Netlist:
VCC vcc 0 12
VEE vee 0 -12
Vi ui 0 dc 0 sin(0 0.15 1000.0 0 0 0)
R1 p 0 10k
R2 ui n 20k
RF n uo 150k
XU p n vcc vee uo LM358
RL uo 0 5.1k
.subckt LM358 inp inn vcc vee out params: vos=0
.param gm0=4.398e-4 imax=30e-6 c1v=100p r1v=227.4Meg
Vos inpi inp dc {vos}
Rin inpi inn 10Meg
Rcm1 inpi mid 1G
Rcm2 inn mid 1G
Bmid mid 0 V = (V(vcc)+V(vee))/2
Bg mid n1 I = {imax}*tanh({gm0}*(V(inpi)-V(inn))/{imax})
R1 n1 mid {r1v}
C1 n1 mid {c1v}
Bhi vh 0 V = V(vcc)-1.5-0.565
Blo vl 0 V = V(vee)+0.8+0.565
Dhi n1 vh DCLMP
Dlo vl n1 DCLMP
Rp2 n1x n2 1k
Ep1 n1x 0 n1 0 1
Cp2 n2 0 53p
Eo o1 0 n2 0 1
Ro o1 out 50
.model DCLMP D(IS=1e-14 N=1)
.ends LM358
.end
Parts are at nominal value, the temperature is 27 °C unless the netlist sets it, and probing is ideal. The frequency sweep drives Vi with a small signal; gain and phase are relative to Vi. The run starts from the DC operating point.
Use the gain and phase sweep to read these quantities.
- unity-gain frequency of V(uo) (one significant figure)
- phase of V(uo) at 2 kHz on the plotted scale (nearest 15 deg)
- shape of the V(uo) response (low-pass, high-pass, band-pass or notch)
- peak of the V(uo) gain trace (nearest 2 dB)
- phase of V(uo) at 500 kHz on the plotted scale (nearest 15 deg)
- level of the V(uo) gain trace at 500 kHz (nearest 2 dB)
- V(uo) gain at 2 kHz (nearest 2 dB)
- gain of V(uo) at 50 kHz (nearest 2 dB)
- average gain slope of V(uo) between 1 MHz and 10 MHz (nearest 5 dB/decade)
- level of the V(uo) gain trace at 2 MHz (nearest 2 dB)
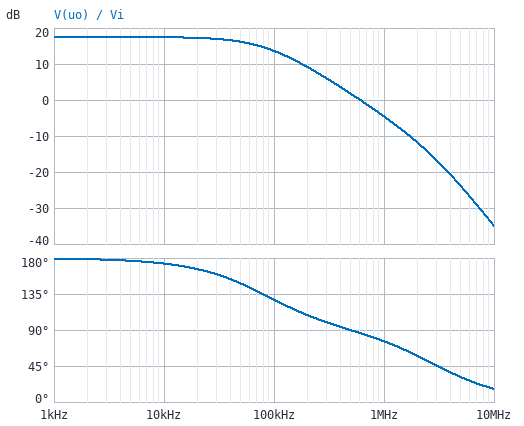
600 kHz
180 deg
low-pass
18 dB
90 deg
2 dB
18 dB
16 dB
-30 dB/decade
-12 dB
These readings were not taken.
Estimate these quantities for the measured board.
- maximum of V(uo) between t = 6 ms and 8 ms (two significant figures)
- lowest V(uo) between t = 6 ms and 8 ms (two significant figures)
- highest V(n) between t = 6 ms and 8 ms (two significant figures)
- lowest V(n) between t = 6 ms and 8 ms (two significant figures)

1.1 V
-1.1 V
1.6 mV
-1.6 mV
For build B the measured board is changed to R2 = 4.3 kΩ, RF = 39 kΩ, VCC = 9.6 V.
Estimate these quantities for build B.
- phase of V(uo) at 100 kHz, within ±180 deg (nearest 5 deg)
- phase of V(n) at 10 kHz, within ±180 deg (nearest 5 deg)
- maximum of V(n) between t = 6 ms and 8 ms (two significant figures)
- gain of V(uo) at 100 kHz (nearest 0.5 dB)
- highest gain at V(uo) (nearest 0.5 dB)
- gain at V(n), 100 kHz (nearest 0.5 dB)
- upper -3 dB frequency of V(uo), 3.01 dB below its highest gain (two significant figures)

125 deg
80 deg
1.9 mV
14.5 dB
19.0 dB
-2.5 dB
70 kHz
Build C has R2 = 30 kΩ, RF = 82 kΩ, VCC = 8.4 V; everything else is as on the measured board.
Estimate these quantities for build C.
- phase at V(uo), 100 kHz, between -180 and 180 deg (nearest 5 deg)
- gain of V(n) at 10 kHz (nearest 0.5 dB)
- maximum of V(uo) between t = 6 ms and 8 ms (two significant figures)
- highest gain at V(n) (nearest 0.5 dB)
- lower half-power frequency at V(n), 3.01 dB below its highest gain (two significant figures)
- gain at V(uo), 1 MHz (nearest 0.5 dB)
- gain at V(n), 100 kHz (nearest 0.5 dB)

150 deg
-28.0 dB
410 mV
-2.5 dB
190 kHz
-6.0 dB
-9.0 dB
